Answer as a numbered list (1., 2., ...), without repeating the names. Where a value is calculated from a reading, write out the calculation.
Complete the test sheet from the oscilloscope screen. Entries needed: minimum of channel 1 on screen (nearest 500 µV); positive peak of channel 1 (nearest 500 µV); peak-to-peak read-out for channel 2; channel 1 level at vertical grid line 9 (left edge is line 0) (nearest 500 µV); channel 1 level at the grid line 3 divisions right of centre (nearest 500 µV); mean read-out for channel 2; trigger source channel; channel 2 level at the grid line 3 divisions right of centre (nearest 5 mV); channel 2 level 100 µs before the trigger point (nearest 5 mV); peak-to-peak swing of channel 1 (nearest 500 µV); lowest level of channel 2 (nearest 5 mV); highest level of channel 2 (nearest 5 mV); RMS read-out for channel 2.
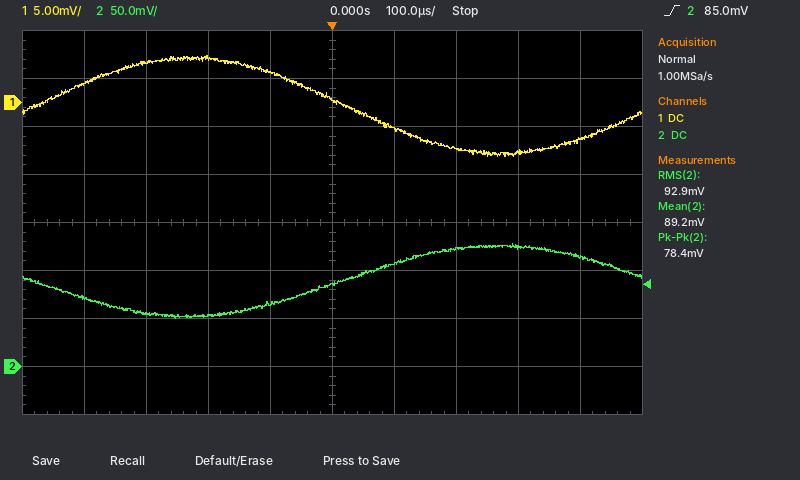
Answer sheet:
1. -5.5 mV
2. 5.0 mV
3. 78.4 mV
4. -4.0 mV
5. -5.0 mV
6. 89.2 mV
7. channel 2
8. 125 mV
9. 65 mV
10. 5.0 mV − (-5.5 mV) = 10.5 mV
11. 50 mV
12. 130 mV
13. 92.9 mV
